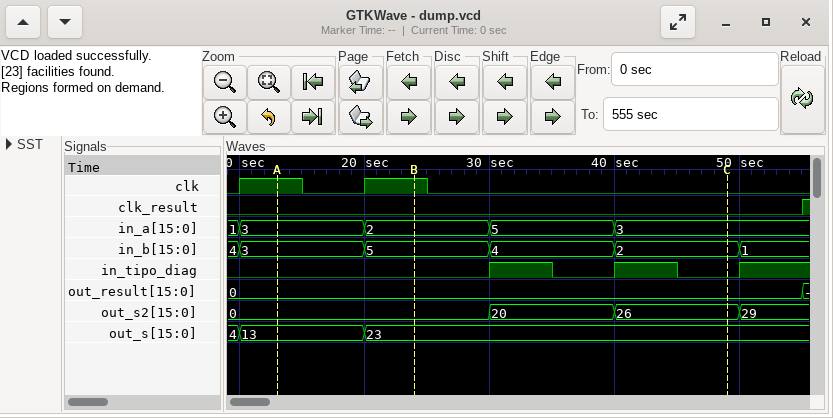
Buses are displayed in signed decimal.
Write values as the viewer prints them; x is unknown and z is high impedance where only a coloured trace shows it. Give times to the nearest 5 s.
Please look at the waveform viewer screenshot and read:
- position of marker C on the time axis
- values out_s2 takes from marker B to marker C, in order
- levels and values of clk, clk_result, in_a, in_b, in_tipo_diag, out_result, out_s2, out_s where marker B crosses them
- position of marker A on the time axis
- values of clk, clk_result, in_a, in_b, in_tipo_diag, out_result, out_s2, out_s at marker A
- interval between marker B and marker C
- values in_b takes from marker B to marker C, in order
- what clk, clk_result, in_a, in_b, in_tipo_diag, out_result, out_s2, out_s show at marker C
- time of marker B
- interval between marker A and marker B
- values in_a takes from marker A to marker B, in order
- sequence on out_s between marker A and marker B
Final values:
50 s
0, 20, 26
clk=1, clk_result=0, in_a=2, in_b=5, in_tipo_diag=0, out_result=0, out_s2=0, out_s=23
15 s
clk=1, clk_result=0, in_a=3, in_b=3, in_tipo_diag=0, out_result=0, out_s2=0, out_s=13
25 s
5, 4, 2
clk=0, clk_result=0, in_a=3, in_b=2, in_tipo_diag=0, out_result=0, out_s2=26, out_s=23
25 s
10 s
3, 2
13, 23
